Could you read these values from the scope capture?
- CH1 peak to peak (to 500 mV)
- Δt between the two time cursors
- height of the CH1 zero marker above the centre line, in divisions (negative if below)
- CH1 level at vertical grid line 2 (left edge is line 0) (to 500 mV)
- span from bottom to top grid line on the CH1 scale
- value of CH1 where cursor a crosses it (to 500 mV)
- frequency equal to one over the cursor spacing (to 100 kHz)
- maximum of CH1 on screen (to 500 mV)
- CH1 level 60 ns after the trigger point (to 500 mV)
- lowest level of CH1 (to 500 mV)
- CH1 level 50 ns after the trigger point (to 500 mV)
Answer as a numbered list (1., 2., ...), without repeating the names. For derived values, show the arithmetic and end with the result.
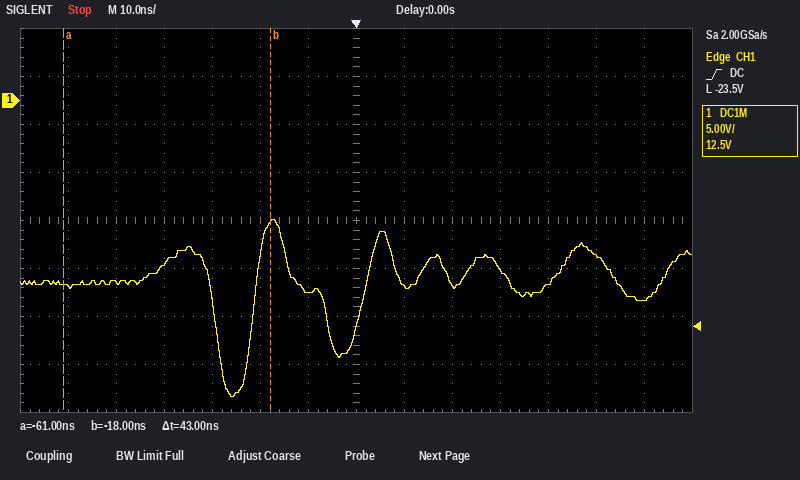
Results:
1. -12.5 V − (-31.0 V) = 18.5 V
2. 43 ns
3. +2.5 div
4. -19.0 V
5. 40 V
6. -19.0 V
7. 1 / 43 ns ≈ 23.3 MHz
8. -12.5 V
9. -21.0 V
10. -31.0 V
11. -16.0 V
